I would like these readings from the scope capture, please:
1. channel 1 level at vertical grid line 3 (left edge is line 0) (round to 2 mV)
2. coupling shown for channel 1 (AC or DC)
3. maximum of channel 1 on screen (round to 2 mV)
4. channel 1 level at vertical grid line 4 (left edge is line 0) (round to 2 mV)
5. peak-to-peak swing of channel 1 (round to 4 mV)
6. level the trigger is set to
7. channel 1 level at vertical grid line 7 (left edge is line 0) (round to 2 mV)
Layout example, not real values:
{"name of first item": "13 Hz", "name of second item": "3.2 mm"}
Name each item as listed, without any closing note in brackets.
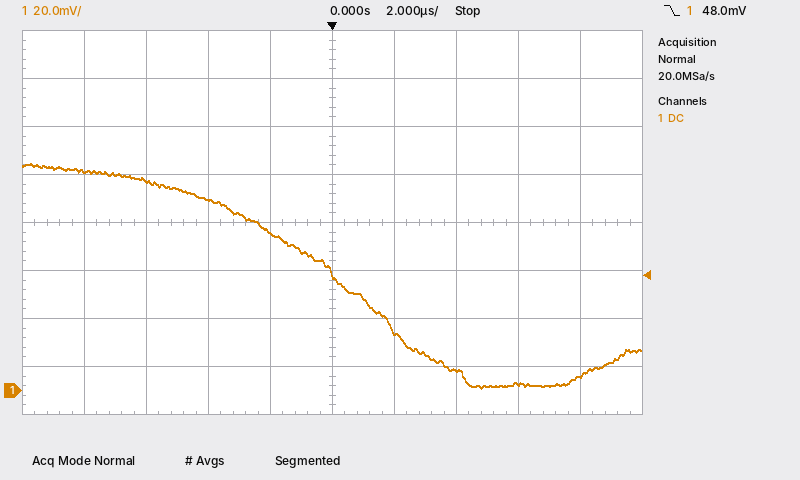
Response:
{"channel 1 level at vertical grid line 3 (left edge is line 0)": "80 mV", "coupling shown for channel 1": "DC", "maximum of channel 1 on screen": "94 mV", "channel 1 level at vertical grid line 4 (left edge is line 0)": "66 mV", "peak-to-peak swing of channel 1": "92 mV", "level the trigger is set to": "48.0 mV", "channel 1 level at vertical grid line 7 (left edge is line 0)": "8 mV"}
